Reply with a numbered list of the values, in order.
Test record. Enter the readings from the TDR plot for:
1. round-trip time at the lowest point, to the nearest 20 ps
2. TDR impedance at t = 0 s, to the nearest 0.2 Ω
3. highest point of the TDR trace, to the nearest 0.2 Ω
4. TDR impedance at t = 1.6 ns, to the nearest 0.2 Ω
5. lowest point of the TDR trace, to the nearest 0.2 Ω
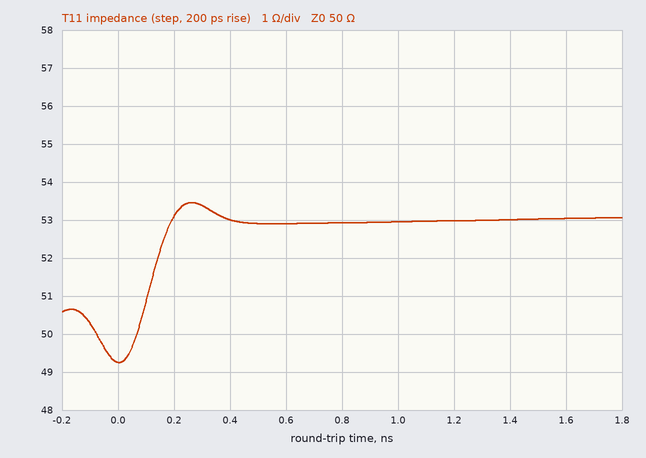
1. 0 ps
2. 49.2 Ω
3. 53.4 Ω
4. 53.0 Ω
5. 49.2 Ω
